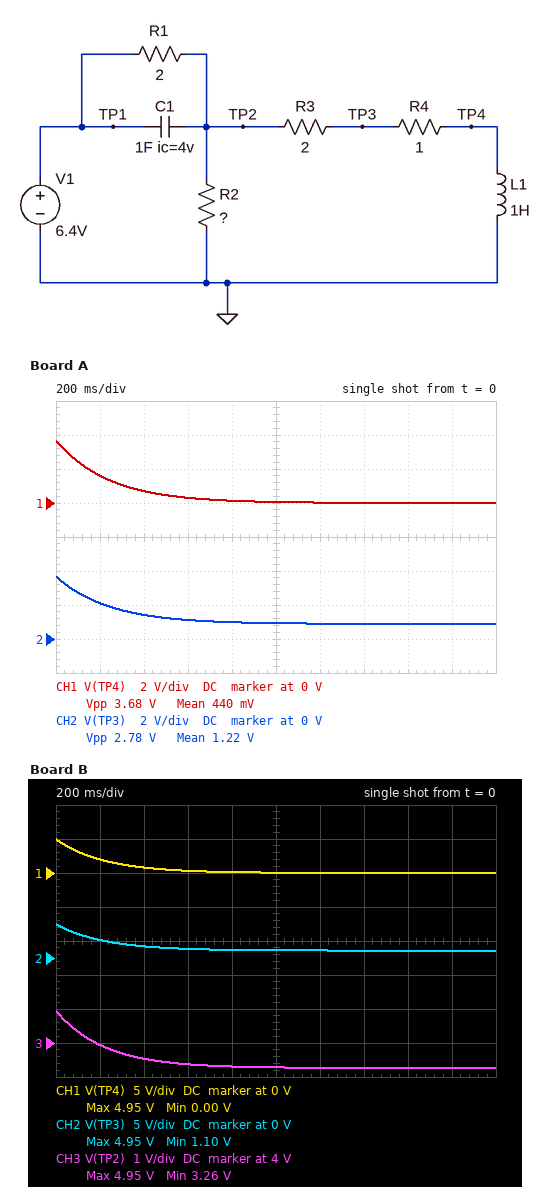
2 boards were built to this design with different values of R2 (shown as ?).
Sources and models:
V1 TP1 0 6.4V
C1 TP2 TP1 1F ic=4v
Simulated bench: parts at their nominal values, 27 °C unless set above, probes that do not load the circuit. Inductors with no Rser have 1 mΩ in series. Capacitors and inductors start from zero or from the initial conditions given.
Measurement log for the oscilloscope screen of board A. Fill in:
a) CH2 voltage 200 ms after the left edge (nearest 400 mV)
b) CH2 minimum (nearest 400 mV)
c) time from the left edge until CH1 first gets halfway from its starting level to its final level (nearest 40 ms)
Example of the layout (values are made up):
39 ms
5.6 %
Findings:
2.0 V
800 mV
160 ms
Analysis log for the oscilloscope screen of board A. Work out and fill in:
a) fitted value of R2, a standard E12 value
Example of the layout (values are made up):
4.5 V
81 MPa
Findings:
2.7 Ω
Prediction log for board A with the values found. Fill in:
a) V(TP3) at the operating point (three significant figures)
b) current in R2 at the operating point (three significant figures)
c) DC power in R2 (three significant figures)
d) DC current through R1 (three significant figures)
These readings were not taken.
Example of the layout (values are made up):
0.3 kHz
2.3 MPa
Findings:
887 mV
985 mA
2.62 W
1.87 A
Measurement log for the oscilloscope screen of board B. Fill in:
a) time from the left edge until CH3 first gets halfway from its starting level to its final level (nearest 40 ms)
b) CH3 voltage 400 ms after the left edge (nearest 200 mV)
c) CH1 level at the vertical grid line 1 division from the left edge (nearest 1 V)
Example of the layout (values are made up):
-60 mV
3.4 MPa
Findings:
160 ms
3.6 V
2 V
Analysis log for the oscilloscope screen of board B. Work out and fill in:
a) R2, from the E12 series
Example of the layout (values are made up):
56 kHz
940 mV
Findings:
6.8 Ω
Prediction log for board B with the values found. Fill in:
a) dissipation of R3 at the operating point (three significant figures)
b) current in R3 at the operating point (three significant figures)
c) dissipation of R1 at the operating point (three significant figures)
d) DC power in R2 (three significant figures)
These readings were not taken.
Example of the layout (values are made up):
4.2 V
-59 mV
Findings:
2.37 W
1.09 A
4.92 W
1.57 W
